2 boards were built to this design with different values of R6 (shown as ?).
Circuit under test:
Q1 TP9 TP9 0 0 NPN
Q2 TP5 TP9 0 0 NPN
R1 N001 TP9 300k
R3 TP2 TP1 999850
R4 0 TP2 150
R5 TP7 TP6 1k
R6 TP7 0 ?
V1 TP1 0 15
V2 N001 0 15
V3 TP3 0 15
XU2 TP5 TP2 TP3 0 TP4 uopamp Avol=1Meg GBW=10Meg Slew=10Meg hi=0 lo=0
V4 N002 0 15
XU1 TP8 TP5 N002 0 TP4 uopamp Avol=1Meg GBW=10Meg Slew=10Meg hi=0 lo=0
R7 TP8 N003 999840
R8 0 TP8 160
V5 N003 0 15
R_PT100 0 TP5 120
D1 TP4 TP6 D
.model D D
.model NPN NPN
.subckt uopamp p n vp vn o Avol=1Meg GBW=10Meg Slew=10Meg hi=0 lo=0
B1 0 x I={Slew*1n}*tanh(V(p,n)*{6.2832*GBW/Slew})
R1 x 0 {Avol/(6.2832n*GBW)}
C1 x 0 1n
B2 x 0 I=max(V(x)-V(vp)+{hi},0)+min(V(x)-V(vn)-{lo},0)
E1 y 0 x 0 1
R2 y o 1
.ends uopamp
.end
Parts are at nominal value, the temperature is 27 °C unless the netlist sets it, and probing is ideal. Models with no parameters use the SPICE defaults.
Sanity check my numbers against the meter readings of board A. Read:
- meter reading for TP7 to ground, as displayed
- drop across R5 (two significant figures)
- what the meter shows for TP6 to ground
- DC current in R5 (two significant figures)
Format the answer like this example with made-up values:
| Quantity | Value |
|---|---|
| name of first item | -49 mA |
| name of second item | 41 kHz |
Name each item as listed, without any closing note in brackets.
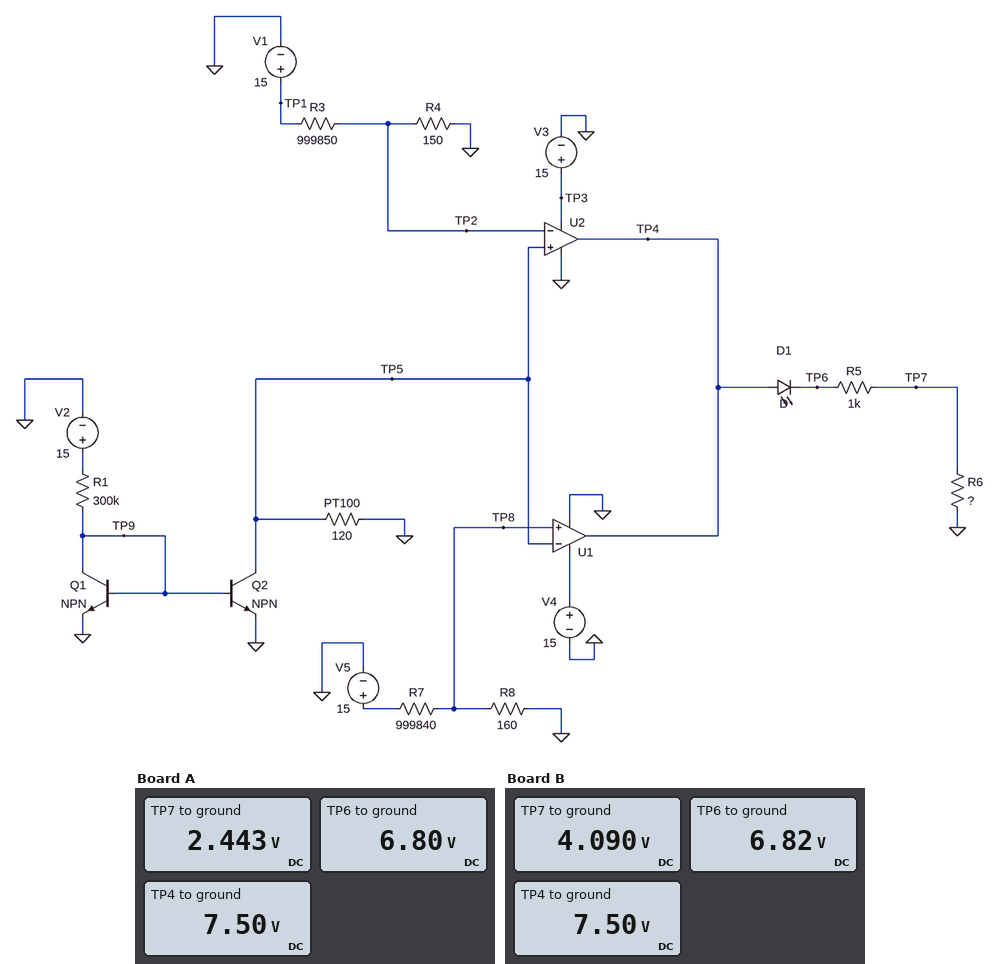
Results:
| Quantity | Value |
|---|---|
| meter reading for TP7 to ground, as displayed | 2.443 V |
| drop across R5 | 4.4 V |
| what the meter shows for TP6 to ground | 6.80 V |
| DC current in R5 | 4.4 mA |
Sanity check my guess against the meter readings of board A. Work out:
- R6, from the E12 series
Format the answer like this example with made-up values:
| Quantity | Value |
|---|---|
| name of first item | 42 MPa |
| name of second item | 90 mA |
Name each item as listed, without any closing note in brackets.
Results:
| Quantity | Value |
|---|---|
| R6, from the E12 series | 560 Ω |
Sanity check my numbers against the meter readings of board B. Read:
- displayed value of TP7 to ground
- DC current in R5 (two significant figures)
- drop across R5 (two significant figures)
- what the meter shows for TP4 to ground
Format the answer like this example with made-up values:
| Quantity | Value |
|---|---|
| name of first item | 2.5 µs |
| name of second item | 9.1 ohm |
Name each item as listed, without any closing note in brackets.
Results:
| Quantity | Value |
|---|---|
| displayed value of TP7 to ground | 4.090 V |
| DC current in R5 | 2.7 mA |
| drop across R5 | 2.7 V |
| what the meter shows for TP4 to ground | 7.50 V |
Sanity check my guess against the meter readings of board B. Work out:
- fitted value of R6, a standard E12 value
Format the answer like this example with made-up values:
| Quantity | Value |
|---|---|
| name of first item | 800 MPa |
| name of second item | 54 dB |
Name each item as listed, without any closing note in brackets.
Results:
| Quantity | Value |
|---|---|
| fitted value of R6, a standard E12 value | 1.5 kΩ |
